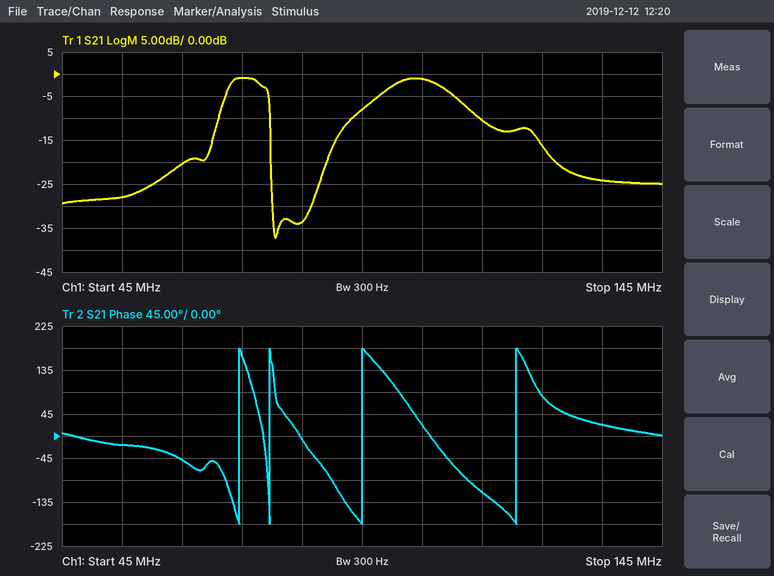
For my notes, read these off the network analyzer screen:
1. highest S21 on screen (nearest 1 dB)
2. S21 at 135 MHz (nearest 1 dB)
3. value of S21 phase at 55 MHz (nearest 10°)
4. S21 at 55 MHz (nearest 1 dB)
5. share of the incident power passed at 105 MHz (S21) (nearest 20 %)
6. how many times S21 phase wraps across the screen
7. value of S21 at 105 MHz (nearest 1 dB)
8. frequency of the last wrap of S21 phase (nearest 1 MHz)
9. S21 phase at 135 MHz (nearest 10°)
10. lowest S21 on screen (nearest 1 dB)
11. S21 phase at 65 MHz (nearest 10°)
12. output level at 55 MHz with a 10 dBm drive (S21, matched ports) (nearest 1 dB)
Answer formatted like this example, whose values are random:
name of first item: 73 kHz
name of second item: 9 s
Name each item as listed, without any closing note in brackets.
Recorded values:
highest S21 on screen: -1 dB
S21 at 135 MHz: -24 dB
value of S21 phase at 55 MHz: -20°
S21 at 55 MHz: -28 dB
share of the incident power passed at 105 MHz (S21): 80 %
how many times S21 phase wraps across the screen: 4
value of S21 at 105 MHz: -1 dB
frequency of the last wrap of S21 phase: 121 MHz
S21 phase at 135 MHz: 20°
lowest S21 on screen: -37 dB
S21 phase at 65 MHz: -50°
output level at 55 MHz with a 10 dBm drive (S21, matched ports): -18 dBm
